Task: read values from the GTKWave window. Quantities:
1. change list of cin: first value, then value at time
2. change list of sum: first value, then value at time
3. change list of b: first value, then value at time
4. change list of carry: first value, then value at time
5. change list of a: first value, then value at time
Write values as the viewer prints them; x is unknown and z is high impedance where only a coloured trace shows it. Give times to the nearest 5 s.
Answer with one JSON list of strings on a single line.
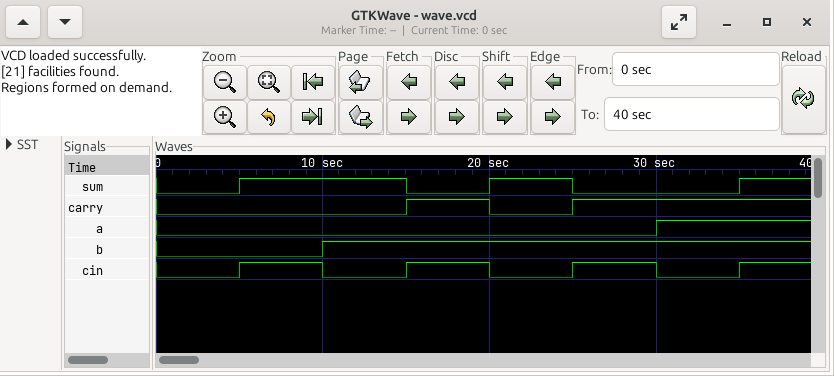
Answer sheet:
["0, 1 at 5 s, 0 at 10 s, 1 at 15 s, 0 at 20 s, 1 at 25 s, 0 at 30 s, 1 at 35 s", "0, 1 at 5 s, 0 at 15 s, 1 at 20 s, 0 at 25 s, 1 at 35 s", "0, 1 at 10 s", "0, 1 at 15 s, 0 at 20 s, 1 at 25 s", "0, 1 at 30 s"]
